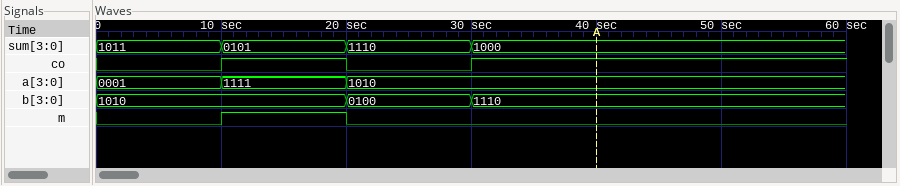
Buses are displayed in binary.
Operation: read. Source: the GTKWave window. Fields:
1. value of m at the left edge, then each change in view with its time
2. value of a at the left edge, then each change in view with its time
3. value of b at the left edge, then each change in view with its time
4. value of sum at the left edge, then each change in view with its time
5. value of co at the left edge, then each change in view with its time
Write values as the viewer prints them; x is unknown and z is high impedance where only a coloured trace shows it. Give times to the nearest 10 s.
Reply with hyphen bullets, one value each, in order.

- 0, 1 at 10 s, 0 at 20 s
- 0001, 1111 at 10 s, 1010 at 20 s
- 1010, 0100 at 20 s, 1110 at 30 s
- 1011, 0101 at 10 s, 1110 at 20 s, 1000 at 30 s
- 0, 1 at 10 s, 0 at 20 s, 1 at 30 s
